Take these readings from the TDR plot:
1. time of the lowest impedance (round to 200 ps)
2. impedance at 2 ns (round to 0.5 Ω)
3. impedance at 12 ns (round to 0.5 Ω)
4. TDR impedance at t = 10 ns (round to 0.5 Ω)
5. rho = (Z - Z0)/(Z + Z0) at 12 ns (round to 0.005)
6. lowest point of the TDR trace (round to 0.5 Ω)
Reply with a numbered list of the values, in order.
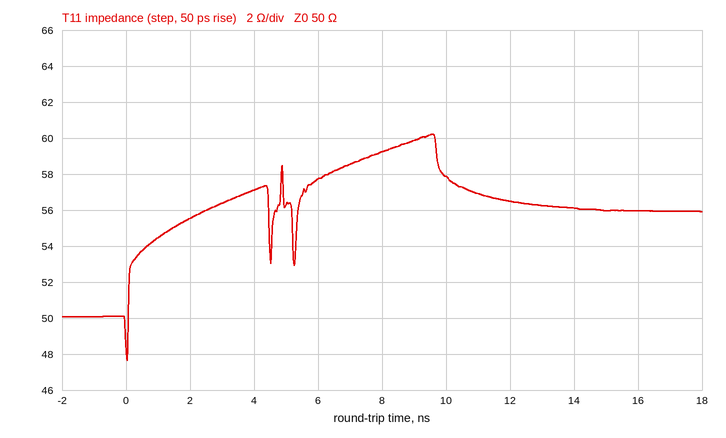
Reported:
1. 0.0 ns
2. 55.5 Ω
3. 56.5 Ω
4. 58.0 Ω
5. +0.060
6. 47.5 Ω
